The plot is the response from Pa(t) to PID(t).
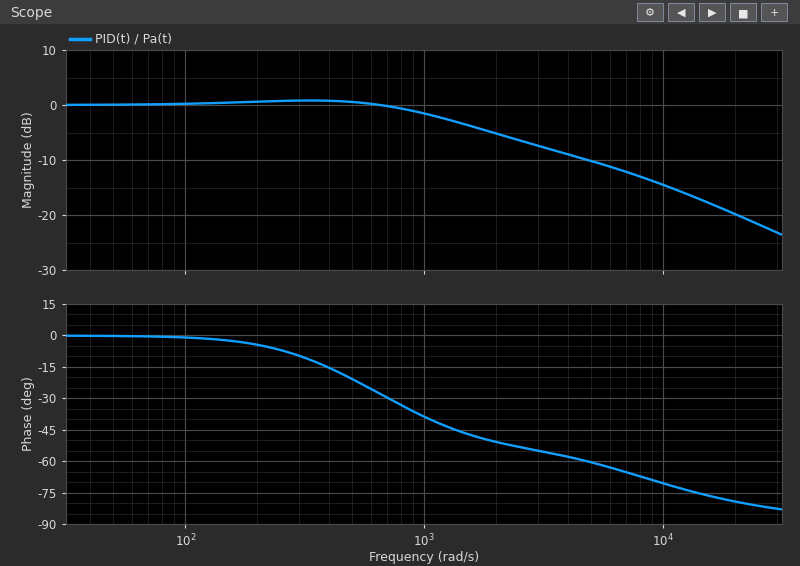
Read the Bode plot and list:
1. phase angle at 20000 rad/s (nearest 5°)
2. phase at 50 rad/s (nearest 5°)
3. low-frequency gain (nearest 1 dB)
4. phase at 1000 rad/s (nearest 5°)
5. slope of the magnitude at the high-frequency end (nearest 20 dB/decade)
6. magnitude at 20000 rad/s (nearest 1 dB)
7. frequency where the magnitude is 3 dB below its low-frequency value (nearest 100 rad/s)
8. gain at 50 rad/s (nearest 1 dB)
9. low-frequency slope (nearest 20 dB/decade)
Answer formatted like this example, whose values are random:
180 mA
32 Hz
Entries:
-80°
0°
0 dB
-40°
-20 dB/decade
-20 dB
1300 rad/s
0 dB
0 dB/decade
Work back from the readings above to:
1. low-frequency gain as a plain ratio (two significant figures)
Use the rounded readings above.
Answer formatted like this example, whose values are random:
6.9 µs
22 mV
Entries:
1.0
